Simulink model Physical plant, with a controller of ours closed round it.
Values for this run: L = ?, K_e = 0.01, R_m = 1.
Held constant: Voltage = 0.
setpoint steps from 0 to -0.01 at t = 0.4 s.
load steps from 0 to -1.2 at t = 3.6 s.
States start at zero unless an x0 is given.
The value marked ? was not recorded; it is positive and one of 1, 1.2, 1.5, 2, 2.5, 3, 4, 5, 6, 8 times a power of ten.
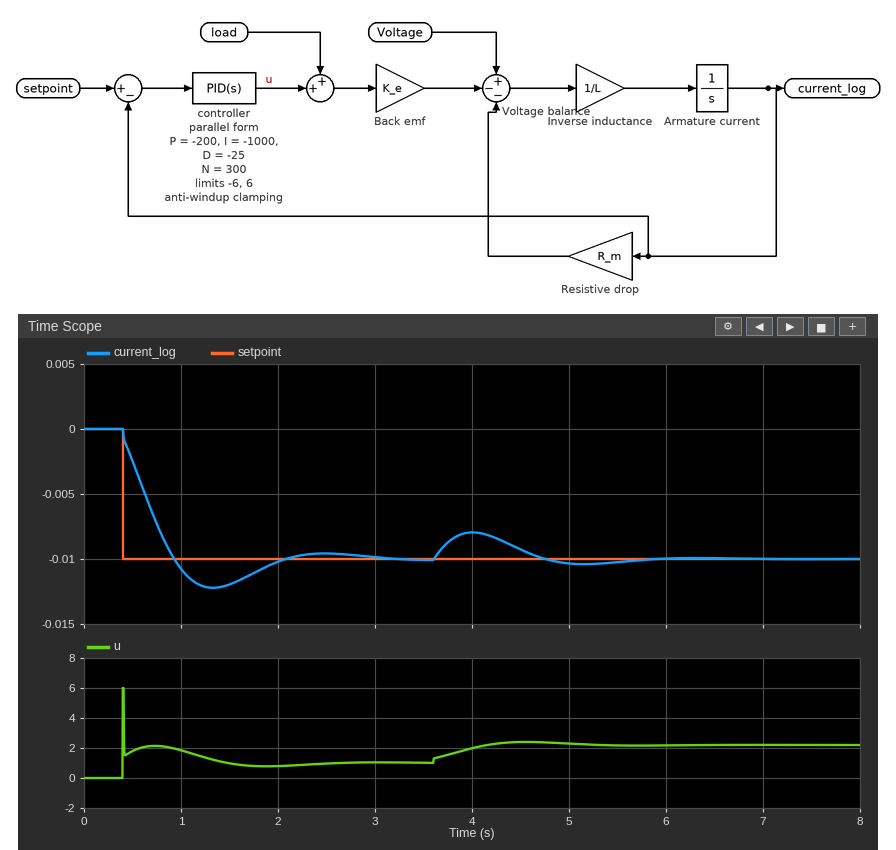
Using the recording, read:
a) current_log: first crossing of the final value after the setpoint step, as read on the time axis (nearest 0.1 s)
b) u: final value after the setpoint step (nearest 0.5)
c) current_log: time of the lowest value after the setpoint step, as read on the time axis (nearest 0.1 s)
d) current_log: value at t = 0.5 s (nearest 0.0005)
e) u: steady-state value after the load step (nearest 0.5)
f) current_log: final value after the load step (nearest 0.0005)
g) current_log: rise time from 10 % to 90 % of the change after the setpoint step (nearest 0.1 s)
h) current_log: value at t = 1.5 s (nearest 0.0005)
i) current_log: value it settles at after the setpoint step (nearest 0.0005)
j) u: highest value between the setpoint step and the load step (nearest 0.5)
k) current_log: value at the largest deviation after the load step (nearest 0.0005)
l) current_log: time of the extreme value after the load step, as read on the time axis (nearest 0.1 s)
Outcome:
0.9 s
1.0
1.3 s
-0.0025
2.0
-0.0100
0.4 s
-0.0120
-0.0100
6.0
-0.0080
4.0 s
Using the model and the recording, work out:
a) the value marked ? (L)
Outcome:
0.8
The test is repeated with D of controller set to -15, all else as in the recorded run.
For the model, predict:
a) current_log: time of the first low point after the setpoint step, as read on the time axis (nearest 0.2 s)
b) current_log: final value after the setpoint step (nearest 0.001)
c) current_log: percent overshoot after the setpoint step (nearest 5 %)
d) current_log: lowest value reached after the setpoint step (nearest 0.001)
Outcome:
1.2 s
-0.010
20 %
-0.012
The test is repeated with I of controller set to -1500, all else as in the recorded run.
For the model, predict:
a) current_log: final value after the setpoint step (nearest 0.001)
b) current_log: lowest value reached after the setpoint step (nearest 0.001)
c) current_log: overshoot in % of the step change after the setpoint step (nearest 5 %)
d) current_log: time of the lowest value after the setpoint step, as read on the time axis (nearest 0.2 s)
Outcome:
-0.010
-0.013
30 %
1.2 s
